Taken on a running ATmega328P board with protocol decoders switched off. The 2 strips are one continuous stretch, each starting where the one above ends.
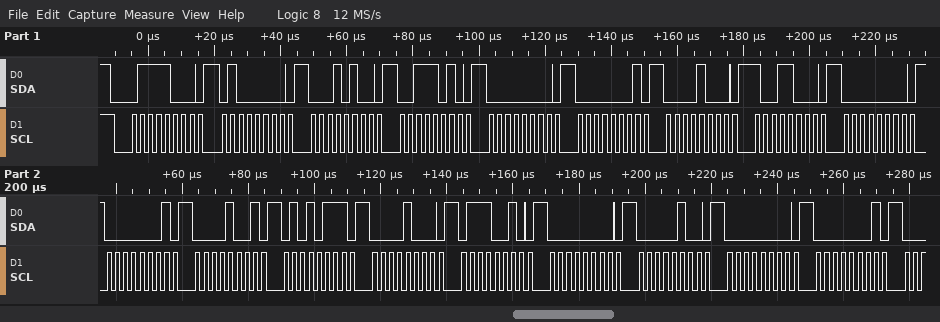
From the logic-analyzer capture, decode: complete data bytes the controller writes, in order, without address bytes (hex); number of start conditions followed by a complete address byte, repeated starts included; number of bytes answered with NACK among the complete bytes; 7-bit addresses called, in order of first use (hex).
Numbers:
40 14 3A 00 01 08 98 00 01 09 57 08 72 00 04 00 01
1
0
0x3C
